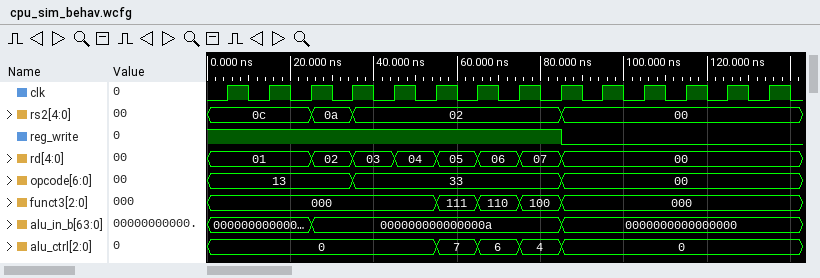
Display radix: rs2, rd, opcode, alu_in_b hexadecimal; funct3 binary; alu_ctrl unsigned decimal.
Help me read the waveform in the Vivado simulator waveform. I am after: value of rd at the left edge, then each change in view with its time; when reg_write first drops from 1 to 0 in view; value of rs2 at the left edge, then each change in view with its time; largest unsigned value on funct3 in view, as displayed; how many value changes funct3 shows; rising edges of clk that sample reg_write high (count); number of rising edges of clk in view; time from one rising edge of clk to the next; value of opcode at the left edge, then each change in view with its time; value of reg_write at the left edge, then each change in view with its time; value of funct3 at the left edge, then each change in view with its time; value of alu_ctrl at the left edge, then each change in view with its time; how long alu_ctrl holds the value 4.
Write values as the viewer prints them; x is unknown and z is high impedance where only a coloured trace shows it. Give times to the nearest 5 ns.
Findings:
01, 02 at 25 ns, 03 at 35 ns, 04 at 45 ns, 05 at 55 ns, 06 at 65 ns, 07 at 75 ns, 00 at 85 ns
85 ns
0c, 0a at 25 ns, 02 at 35 ns, 00 at 85 ns
111
4
9
14
10 ns
13, 33 at 35 ns, 00 at 85 ns
1, 0 at 85 ns
000, 111 at 55 ns, 110 at 65 ns, 100 at 75 ns, 000 at 85 ns
0, 7 at 55 ns, 6 at 65 ns, 4 at 75 ns, 0 at 85 ns
10 ns
